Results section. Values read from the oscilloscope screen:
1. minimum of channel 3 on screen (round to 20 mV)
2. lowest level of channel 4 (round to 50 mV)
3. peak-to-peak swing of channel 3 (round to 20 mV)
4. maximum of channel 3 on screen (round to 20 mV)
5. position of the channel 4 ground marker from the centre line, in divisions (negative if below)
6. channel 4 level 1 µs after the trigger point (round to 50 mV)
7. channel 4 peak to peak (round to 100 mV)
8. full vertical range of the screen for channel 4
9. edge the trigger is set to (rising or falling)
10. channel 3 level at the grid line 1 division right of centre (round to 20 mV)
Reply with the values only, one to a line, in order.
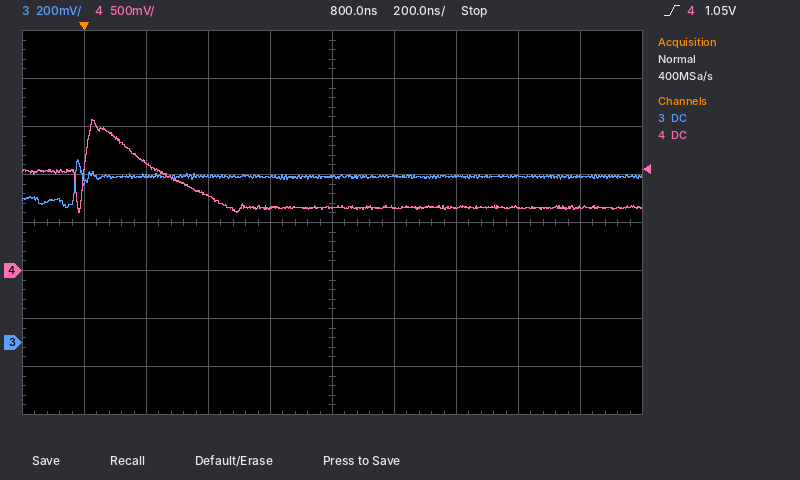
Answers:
560 mV
600 mV
200 mV
760 mV
-1.0 div
650 mV
1.00 V
4 V
rising
700 mV
